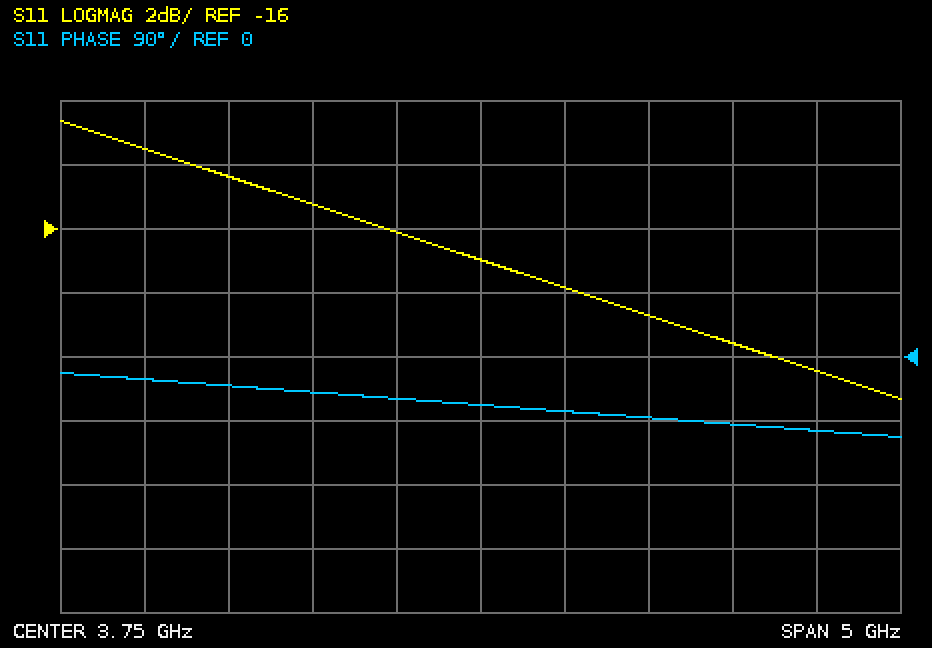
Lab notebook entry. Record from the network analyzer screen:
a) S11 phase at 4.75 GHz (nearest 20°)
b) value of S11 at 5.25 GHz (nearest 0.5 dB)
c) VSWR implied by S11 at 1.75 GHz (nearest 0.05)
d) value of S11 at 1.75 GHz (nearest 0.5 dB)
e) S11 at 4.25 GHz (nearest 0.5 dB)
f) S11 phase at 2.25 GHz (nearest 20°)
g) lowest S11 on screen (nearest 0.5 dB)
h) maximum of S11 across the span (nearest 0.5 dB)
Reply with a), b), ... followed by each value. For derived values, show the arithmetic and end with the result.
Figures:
a) -80°
b) -19.5 dB
c) |Γ| = 10^(-13.5/20) = 0.2113; VSWR = (1 + 0.2113)/(1 − 0.2113) ≈ 1.54, so 1.55 to the nearest 0.05
d) -13.5 dB
e) -18.0 dB
f) -40°
g) -21.5 dB
h) -12.5 dB
